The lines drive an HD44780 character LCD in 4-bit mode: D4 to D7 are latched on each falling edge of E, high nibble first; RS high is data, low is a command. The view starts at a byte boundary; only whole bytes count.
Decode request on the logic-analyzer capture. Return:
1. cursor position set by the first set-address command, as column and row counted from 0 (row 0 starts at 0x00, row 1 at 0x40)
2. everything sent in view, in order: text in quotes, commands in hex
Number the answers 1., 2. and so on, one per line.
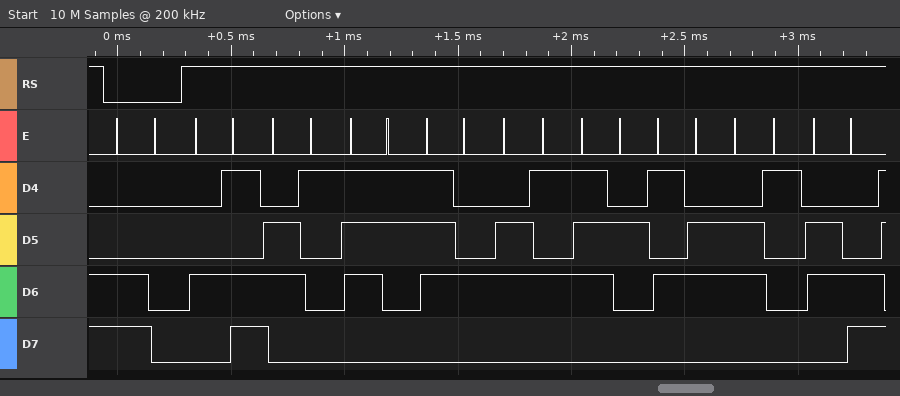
1. column 0, row 1
2. 0xC0 "MasterVal"
